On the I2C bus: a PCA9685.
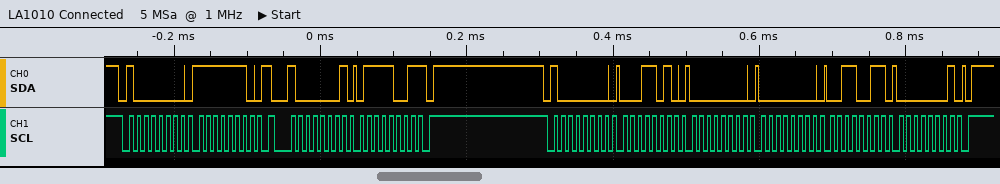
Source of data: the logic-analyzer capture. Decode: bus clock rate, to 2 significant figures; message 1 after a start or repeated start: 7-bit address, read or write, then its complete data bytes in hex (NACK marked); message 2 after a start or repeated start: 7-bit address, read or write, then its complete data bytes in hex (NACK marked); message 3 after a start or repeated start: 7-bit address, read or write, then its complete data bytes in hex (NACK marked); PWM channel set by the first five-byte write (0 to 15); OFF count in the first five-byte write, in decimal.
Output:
100 kHz
0x40 write: FE
0x40 read: 79 NACK
0x40 write: 1A 00 00 33 01
5
307
